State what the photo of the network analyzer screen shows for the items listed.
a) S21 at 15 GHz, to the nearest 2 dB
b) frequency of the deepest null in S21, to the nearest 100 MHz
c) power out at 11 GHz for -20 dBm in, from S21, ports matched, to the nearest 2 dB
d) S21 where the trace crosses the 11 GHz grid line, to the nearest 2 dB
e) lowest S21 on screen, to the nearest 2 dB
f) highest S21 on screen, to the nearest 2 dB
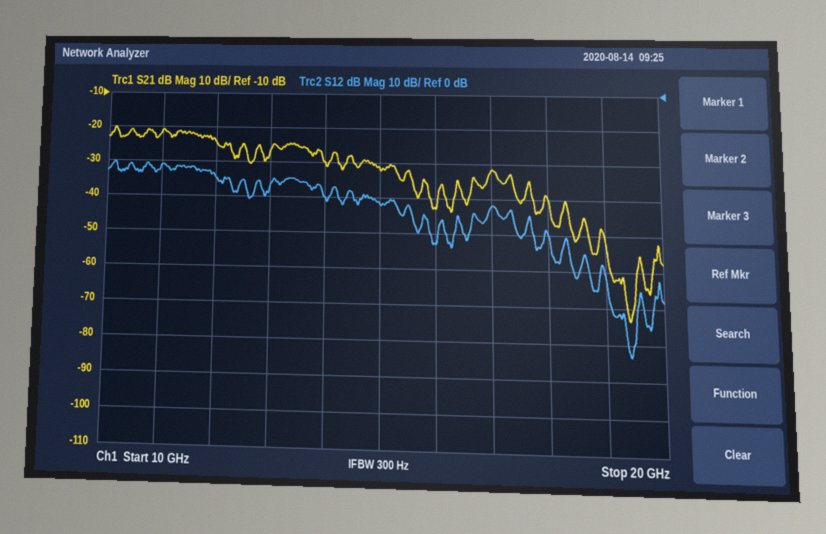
-32 dB
19.4 GHz
-42 dBm
-22 dB
-74 dB
-20 dB
